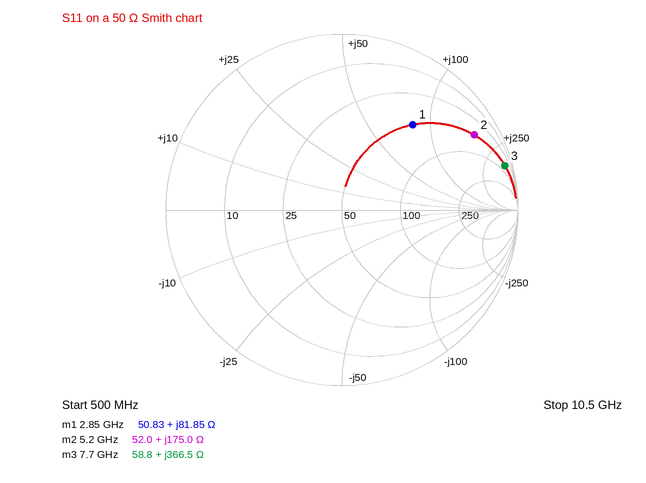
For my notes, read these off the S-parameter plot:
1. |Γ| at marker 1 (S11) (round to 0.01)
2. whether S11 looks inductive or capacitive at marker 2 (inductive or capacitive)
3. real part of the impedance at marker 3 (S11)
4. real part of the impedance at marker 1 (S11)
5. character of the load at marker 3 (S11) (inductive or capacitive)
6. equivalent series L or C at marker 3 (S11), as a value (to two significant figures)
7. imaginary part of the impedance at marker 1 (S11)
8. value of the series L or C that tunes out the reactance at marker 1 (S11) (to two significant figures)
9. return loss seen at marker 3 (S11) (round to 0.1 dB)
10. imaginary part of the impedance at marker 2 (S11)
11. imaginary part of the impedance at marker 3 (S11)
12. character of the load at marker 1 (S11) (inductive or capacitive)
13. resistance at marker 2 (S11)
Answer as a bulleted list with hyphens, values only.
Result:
- 0.63
- inductive
- 58.8 Ω
- 50.83 Ω
- inductive
- 7.6 nH
- +81.85 Ω
- 680 fF
- 0.4 dB
- +175.0 Ω
- +366.5 Ω
- inductive
- 52.0 Ω
